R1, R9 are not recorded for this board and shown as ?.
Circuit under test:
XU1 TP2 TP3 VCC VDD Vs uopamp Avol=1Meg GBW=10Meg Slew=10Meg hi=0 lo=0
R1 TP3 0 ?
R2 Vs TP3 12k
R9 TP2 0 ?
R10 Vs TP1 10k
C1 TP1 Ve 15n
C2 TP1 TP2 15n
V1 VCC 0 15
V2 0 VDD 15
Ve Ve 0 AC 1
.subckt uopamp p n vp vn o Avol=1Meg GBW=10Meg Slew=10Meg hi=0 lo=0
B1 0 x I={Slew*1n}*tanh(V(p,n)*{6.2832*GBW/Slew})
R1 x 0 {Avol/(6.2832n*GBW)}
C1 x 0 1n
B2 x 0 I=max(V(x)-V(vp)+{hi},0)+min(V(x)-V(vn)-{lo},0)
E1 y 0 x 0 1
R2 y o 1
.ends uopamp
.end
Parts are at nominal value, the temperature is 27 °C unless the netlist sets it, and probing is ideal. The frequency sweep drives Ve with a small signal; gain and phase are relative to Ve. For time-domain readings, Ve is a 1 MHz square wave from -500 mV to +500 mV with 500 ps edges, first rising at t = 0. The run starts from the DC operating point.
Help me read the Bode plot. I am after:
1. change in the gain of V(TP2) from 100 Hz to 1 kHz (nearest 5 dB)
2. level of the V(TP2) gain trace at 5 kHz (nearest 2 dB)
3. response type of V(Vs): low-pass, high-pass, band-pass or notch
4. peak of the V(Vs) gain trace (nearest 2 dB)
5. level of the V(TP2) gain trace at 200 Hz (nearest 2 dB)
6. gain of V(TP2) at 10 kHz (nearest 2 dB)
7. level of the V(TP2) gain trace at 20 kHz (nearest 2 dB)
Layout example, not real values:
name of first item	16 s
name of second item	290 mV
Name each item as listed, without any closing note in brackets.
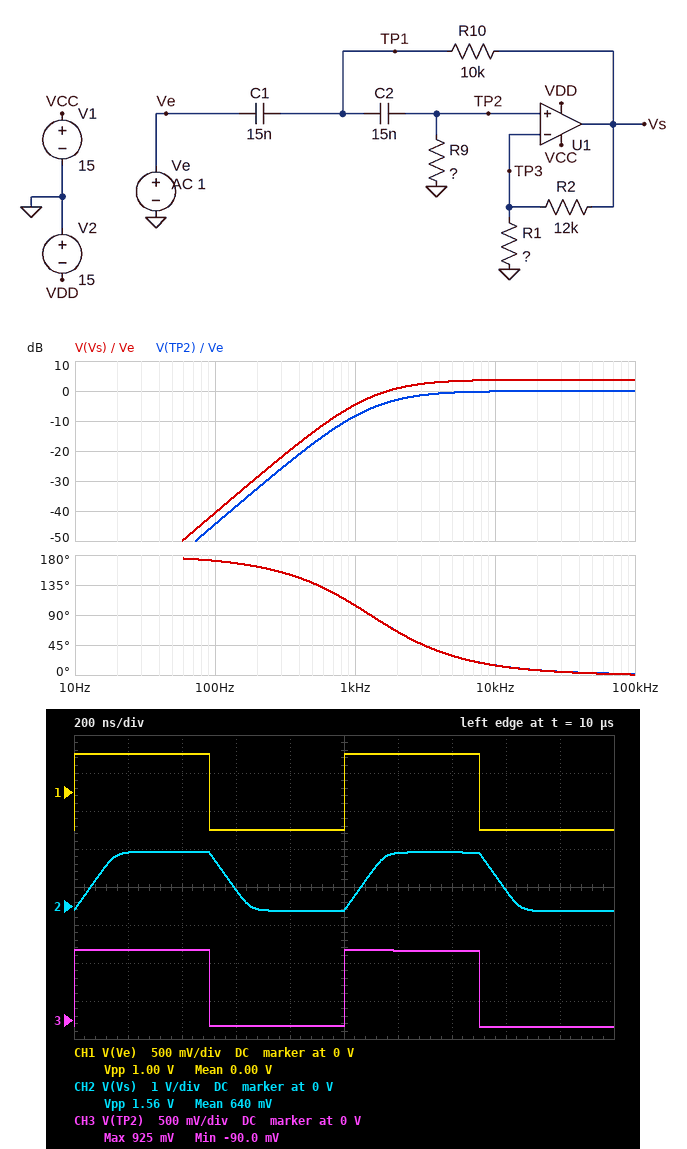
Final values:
change in the gain of V(TP2) from 100 Hz to 1 kHz	35 dB
level of the V(TP2) gain trace at 5 kHz	0 dB
response type of V(Vs): low-pass, high-pass, band-pass or notch	high-pass
peak of the V(Vs) gain trace	4 dB
level of the V(TP2) gain trace at 200 Hz	-32 dB
gain of V(TP2) at 10 kHz	0 dB
level of the V(TP2) gain trace at 20 kHz	0 dB
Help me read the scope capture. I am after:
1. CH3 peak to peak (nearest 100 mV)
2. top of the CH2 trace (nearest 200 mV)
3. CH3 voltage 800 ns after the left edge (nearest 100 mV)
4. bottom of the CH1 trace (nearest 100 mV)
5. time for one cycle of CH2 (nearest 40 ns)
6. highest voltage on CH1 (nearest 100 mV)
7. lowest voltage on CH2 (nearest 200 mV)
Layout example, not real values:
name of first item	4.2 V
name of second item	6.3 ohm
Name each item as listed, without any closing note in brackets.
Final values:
CH3 peak to peak	1.0 V
top of the CH2 trace	1.4 V
CH3 voltage 800 ns after the left edge	-100 mV
bottom of the CH1 trace	-500 mV
time for one cycle of CH2	1.00 µs
highest voltage on CH1	500 mV
lowest voltage on CH2	-200 mV
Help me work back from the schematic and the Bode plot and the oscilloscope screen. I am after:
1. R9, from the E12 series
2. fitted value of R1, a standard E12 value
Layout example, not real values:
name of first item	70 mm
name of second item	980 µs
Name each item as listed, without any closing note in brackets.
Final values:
R9, from the E12 series	6.8 kΩ
fitted value of R1, a standard E12 value	22 kΩ
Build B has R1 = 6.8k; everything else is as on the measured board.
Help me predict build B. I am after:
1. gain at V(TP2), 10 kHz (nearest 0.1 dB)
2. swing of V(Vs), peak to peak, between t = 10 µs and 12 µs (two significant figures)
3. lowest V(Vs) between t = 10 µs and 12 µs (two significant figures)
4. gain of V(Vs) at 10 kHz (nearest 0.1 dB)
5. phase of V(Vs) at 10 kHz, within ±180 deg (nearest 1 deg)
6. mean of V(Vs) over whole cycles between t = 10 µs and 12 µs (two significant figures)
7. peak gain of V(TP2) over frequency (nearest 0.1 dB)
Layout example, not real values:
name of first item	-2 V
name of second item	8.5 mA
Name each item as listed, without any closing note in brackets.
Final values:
gain at V(TP2), 10 kHz	0.1 dB
swing of V(Vs), peak to peak, between t = 10 µs and 12 µs	2.8 V
lowest V(Vs) between t = 10 µs and 12 µs	-130 mV
gain of V(Vs) at 10 kHz	8.9 dB
phase of V(Vs) at 10 kHz, within ±180 deg	7 deg
mean of V(Vs) over whole cycles between t = 10 µs and 12 µs	1.3 V
peak gain of V(TP2) over frequency	1.4 dB
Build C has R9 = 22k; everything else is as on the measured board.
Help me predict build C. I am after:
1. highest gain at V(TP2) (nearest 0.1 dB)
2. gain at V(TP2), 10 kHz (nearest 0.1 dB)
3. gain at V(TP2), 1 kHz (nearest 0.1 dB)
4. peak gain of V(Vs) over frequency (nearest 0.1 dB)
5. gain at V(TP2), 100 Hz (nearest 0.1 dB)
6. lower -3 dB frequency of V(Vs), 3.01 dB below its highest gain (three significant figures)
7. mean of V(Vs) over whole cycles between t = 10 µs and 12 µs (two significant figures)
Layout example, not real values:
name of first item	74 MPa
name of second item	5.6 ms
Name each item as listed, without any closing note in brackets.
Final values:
highest gain at V(TP2)	5.7 dB
gain at V(TP2), 10 kHz	0 dB
gain at V(TP2), 1 kHz	4.1 dB
peak gain of V(Vs) over frequency	9.5 dB
gain at V(TP2), 100 Hz	-34.0 dB
lower -3 dB frequency of V(Vs), 3.01 dB below its highest gain	610 Hz
mean of V(Vs) over whole cycles between t = 10 µs and 12 µs	750 mV
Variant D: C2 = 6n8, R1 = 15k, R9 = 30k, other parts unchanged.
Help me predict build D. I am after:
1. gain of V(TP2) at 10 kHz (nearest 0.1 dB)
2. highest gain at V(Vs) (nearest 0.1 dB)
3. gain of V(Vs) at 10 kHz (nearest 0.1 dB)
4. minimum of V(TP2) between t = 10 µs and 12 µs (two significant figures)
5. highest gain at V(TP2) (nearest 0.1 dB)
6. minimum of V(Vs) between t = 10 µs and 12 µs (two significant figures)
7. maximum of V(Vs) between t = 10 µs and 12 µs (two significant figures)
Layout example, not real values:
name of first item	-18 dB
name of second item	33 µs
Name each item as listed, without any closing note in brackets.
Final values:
gain of V(TP2) at 10 kHz	0.1 dB
highest gain at V(Vs)	15.3 dB
gain of V(Vs) at 10 kHz	5.2 dB
minimum of V(TP2) between t = 10 µs and 12 µs	-13 mV
highest gain at V(TP2)	10.2 dB
minimum of V(Vs) between t = 10 µs and 12 µs	-21 mV
maximum of V(Vs) between t = 10 µs and 12 µs	1.8 V
